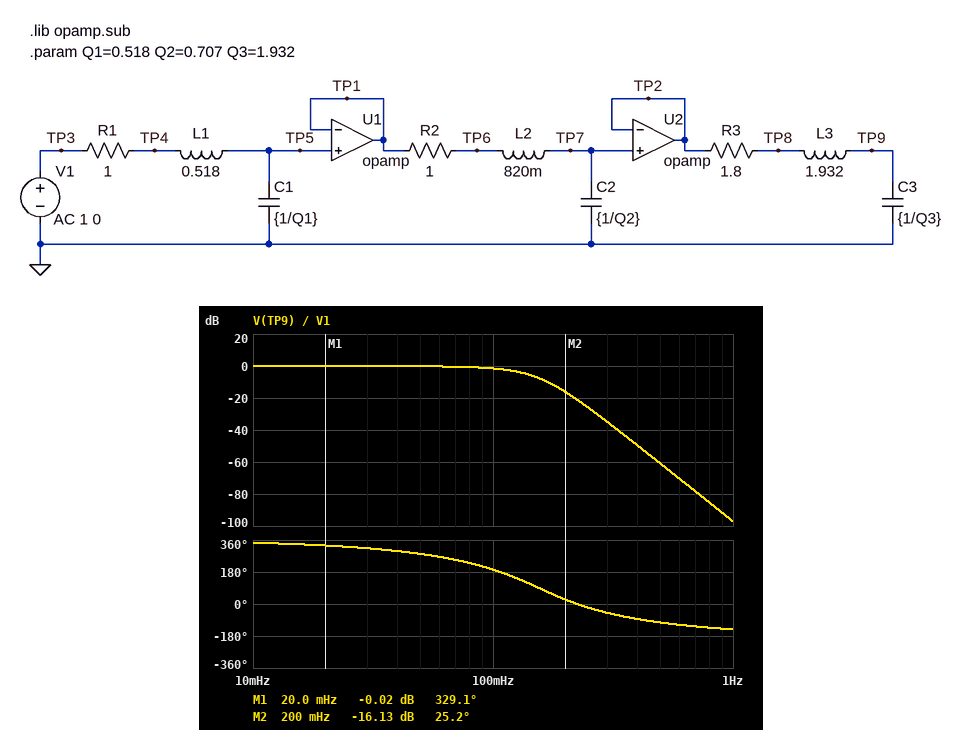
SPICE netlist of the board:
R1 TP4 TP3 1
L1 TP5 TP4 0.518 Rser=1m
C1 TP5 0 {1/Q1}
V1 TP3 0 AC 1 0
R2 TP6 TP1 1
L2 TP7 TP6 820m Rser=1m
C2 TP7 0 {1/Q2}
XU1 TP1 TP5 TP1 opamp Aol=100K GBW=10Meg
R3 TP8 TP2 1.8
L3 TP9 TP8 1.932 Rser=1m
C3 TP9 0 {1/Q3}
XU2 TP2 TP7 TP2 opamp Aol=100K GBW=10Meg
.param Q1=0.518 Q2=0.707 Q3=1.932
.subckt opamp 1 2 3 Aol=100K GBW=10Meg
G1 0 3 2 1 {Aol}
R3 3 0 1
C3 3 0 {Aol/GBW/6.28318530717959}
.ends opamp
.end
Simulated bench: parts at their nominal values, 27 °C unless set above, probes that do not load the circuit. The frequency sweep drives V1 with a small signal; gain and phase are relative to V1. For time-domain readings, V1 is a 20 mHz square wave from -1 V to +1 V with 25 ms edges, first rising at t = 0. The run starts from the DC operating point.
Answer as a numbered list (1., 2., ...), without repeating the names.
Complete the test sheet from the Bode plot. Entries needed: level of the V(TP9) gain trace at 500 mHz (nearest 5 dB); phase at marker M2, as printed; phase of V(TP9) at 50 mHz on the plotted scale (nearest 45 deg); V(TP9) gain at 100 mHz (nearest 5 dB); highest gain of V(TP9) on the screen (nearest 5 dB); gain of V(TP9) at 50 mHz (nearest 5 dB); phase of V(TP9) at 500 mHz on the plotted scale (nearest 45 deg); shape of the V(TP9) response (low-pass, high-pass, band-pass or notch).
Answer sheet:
1. -60 dB
2. 25.2 deg
3. 270 deg
4. 0 dB
5. 0 dB
6. 0 dB
7. -90 deg
8. low-pass
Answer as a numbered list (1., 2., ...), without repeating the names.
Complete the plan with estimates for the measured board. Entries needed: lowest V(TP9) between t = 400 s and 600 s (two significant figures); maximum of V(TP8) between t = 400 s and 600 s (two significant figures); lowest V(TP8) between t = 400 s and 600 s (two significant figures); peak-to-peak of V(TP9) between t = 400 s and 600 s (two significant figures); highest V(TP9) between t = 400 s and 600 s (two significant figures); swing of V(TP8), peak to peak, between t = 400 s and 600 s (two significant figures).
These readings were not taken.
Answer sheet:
1. -1.2 V
2. 1.1 V
3. -1.1 V
4. 2.3 V
5. 1.2 V
6. 2.2 V
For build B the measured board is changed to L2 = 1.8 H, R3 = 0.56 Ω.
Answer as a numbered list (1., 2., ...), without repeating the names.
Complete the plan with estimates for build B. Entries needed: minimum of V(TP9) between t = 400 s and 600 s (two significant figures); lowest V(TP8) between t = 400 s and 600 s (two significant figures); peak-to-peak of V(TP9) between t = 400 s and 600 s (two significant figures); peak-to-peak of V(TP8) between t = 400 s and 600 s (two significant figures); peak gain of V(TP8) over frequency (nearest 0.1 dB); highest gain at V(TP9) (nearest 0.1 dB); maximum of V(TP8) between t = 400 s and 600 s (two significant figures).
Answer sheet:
1. -1.7 V
2. -1.3 V
3. 3.3 V
4. 2.7 V
5. 0.5 dB
6. 2.6 dB
7. 1.3 V
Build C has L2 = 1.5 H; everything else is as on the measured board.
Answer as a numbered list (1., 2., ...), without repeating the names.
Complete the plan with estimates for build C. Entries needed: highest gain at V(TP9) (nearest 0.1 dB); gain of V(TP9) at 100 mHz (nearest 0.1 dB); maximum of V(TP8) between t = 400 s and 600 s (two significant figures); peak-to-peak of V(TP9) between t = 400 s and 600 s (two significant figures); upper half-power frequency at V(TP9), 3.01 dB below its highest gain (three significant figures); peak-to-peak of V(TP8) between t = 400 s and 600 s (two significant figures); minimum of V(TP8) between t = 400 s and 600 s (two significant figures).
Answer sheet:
1. 0.8 dB
2. -0.3 dB
3. 1.2 V
4. 2.7 V
5. 117 mHz
6. 2.4 V
7. -1.2 V
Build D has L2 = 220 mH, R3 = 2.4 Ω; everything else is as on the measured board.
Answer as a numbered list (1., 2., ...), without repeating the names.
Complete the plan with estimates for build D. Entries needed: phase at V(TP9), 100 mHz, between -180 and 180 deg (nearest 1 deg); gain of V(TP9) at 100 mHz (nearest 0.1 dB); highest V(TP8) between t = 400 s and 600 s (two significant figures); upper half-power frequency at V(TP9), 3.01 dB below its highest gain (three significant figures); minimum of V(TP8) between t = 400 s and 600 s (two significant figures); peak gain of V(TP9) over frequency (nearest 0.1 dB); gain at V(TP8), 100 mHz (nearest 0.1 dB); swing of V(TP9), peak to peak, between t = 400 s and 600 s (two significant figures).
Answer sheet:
1. -161 deg
2. -4.5 dB
3. 1.0 V
4. 82.1 mHz
5. -1.0 V
6. 0 dB
7. -8.8 dB
8. 2.0 V
